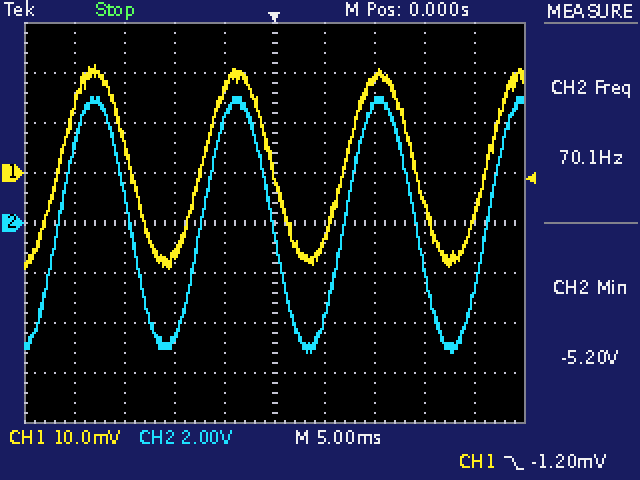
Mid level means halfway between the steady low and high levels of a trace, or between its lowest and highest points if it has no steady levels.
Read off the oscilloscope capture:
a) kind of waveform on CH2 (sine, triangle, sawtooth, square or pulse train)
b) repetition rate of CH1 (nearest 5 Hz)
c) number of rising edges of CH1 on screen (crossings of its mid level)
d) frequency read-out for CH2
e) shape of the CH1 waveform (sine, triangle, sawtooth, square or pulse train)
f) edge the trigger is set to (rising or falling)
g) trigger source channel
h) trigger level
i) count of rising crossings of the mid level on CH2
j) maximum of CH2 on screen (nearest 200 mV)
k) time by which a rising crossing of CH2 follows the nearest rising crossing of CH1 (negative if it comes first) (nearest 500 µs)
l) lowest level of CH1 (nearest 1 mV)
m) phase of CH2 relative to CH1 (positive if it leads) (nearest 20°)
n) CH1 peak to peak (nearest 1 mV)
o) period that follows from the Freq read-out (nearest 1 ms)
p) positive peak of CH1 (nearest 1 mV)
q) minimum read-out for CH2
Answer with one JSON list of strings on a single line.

["sine", "70 Hz", "4", "70.1 Hz", "sine", "falling", "CH1", "-1.20 mV", "4", "5.0 V", "0.0 ms", "-19 mV", "0°", "41 mV", "14 ms", "22 mV", "-5.20 V"]
